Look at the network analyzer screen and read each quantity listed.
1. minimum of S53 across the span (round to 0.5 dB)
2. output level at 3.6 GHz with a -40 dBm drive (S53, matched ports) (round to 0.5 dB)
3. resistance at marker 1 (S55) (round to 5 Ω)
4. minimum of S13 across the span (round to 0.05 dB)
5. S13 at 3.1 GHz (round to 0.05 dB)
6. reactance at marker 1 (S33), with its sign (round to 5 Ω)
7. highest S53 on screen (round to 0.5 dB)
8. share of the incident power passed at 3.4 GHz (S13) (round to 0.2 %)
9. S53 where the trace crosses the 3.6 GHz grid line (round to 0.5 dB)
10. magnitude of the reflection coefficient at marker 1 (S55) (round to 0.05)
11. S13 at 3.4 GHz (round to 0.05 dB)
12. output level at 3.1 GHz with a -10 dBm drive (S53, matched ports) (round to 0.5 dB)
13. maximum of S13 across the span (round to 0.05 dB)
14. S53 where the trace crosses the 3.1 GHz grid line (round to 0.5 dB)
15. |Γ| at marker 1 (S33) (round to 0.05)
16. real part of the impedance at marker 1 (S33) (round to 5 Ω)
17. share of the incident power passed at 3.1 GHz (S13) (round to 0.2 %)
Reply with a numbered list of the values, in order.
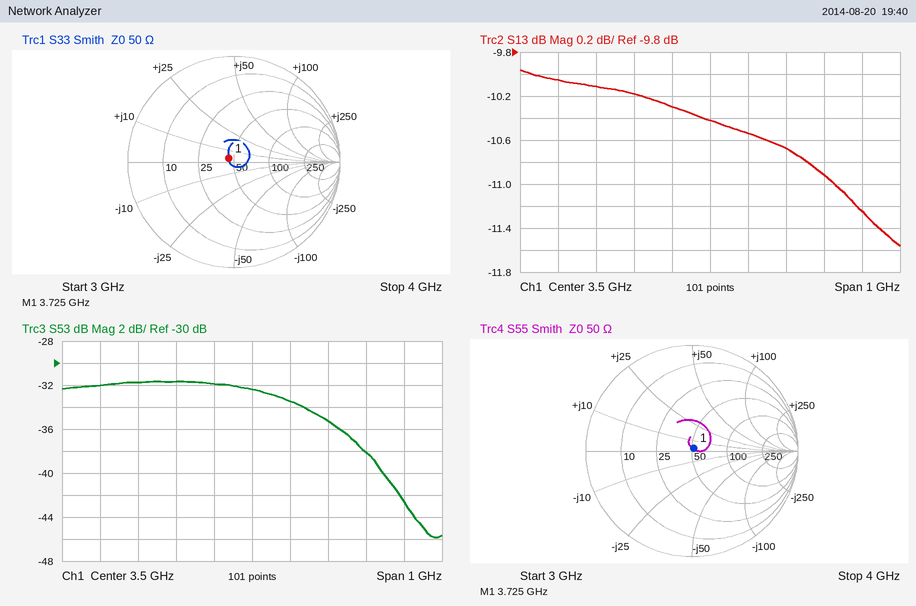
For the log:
1. -46.0 dB
2. -73.5 dBm
3. 50 Ω
4. -11.55 dB
5. -10.05 dB
6. +5 Ω
7. -31.5 dB
8. 9.4 %
9. -33.5 dB
10. 0.05
11. -10.30 dB
12. -42.0 dBm
13. -9.95 dB
14. -32.0 dB
15. 0.05
16. 45 Ω
17. 9.8 %
